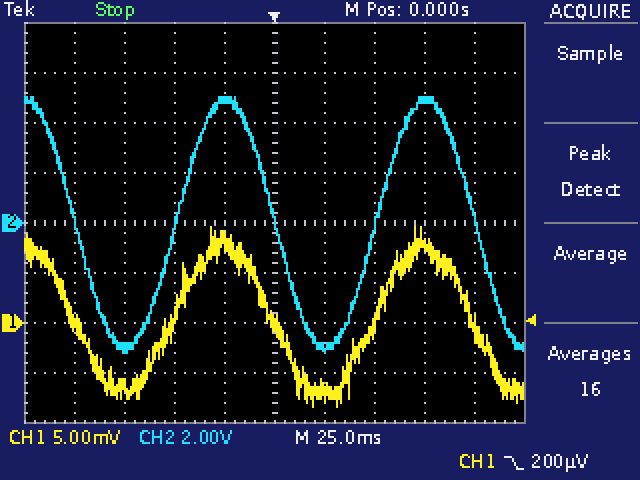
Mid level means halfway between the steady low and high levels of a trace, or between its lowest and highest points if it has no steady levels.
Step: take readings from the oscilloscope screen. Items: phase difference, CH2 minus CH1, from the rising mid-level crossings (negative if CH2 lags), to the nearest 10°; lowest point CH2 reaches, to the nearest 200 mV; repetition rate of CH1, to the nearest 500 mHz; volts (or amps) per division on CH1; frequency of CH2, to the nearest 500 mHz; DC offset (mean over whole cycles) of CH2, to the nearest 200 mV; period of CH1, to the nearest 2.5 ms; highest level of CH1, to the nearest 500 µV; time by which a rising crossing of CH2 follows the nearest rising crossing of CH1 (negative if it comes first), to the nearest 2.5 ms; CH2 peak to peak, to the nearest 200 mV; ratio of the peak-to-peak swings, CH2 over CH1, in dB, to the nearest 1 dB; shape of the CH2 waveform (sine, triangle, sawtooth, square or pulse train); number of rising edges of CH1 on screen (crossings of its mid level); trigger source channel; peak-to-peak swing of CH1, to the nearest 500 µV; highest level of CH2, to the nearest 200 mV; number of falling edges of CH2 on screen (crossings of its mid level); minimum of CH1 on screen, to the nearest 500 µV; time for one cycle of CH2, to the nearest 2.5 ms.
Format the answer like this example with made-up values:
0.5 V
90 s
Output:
0°
-5.2 V
10.0 Hz
5 mV
10.0 Hz
0.0 V
100.0 ms
9.5 mV
0.0 ms
10.2 V
55 dB
sine
2
CH1
18.0 mV
5.0 V
3
-8.5 mV
100.0 ms
